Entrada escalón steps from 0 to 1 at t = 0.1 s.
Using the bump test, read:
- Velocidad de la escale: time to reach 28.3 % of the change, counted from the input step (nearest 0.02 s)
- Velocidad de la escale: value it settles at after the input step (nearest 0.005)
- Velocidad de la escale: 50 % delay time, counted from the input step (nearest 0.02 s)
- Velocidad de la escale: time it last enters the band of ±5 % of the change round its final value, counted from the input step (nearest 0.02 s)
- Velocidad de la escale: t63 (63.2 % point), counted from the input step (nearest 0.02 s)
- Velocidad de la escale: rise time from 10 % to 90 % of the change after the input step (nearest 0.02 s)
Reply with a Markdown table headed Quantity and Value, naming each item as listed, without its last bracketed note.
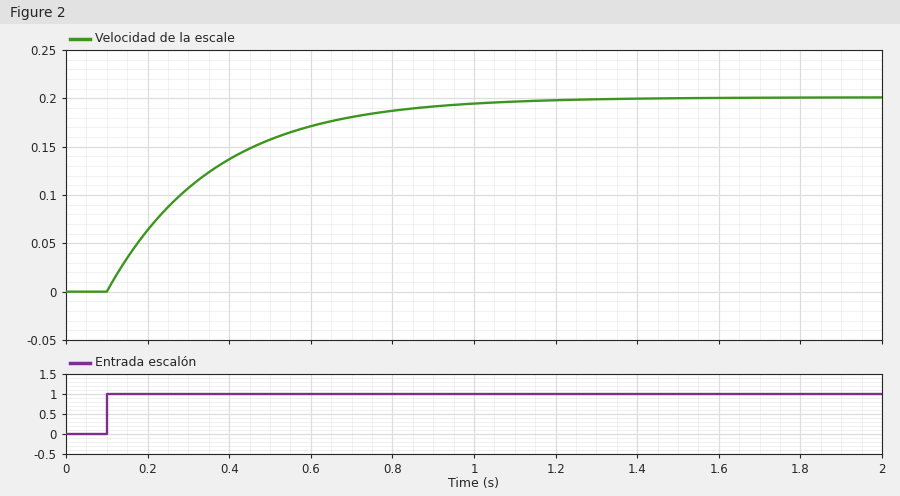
| Quantity | Value |
|---|---|
| Velocidad de la escale: time to reach 28.3 % of the change, counted from the input step | 0.08 s |
| Velocidad de la escale: value it settles at after the input step | 0.200 |
| Velocidad de la escale: 50 % delay time, counted from the input step | 0.18 s |
| Velocidad de la escale: time it last enters the band of ±5 % of the change round its final value, counted from the input step | 0.78 s |
| Velocidad de la escale: t63 (63.2 % point), counted from the input step | 0.26 s |
| Velocidad de la escale: rise time from 10 % to 90 % of the change after the input step | 0.58 s |
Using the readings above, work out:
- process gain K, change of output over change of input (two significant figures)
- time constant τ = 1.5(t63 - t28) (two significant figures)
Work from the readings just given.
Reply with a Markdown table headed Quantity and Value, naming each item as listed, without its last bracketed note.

| Quantity | Value |
|---|---|
| process gain K, change of output over change of input | 0.20 |
| time constant τ = 1.5(t63 - t28) | 0.27 s |
